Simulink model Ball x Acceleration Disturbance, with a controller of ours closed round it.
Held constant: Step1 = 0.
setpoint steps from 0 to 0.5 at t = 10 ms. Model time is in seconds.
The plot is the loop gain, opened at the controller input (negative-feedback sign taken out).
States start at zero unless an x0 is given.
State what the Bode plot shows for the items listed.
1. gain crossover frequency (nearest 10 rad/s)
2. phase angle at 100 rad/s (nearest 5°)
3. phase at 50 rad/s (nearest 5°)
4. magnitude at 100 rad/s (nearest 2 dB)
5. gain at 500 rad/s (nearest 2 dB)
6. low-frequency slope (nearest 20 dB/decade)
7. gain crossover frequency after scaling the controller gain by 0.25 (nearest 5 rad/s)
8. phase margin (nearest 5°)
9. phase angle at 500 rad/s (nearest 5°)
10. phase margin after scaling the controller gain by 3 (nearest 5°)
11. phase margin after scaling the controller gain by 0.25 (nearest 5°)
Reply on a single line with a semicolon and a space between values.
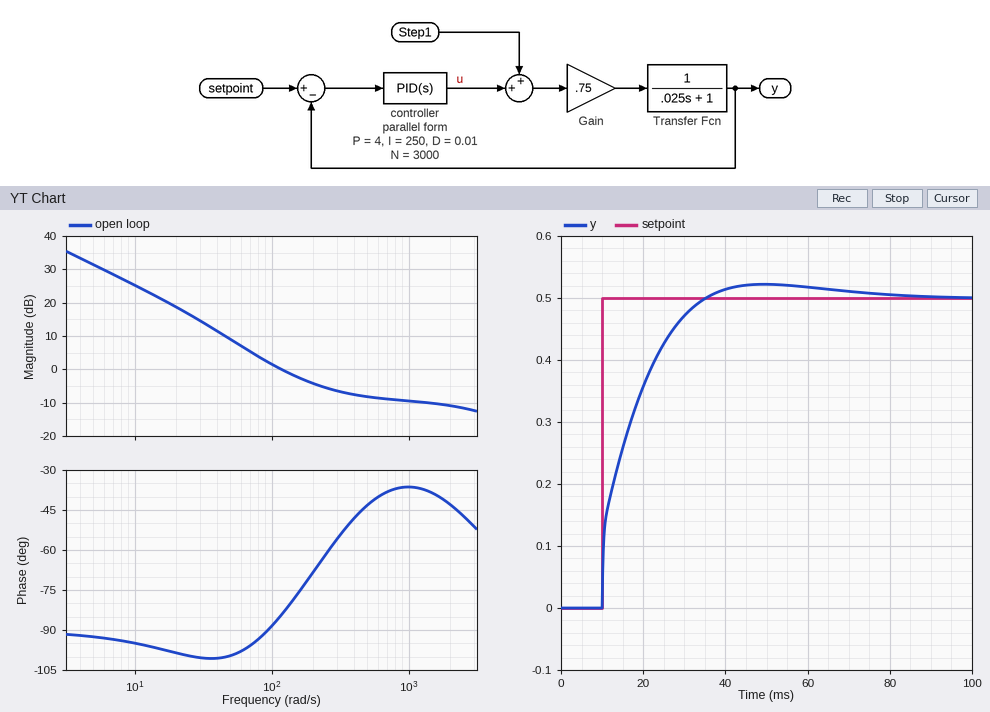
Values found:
120 rad/s; -90°; -100°; 2 dB; -8 dB; -20 dB/decade; 40 rad/s; 95°; -45°; 145°; 80°
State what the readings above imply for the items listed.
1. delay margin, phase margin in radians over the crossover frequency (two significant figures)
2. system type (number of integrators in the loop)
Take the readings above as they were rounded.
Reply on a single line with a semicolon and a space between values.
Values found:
0.014 s; 1
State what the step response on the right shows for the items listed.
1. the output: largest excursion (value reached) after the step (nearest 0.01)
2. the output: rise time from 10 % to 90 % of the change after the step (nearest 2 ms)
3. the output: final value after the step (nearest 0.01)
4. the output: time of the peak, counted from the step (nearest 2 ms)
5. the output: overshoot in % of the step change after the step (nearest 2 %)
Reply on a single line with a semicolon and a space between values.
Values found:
0.52; 18 ms; 0.50; 40 ms; 4 %
